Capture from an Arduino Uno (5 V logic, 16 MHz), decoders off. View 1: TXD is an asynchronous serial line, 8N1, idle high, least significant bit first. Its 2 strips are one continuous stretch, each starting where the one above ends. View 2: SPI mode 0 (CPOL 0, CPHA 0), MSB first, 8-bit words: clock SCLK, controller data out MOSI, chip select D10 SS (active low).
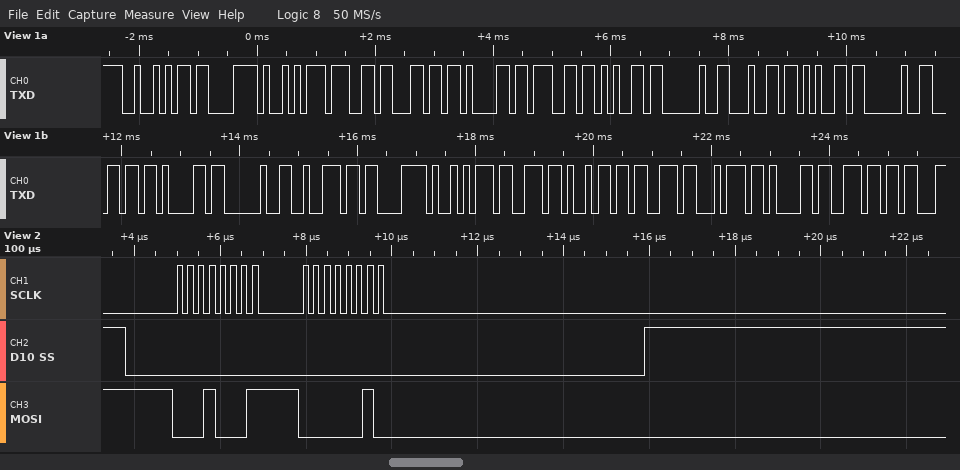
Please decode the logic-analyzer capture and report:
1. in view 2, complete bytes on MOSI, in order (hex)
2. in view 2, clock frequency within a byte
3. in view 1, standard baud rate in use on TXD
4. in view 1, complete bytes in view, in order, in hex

11 02
4 MHz
9600 baud
52 C3 A9 67 6C 61 67 65 20 64 65 20 6C 61 20 72 C3 A9 73 69 73 74 61 6E
